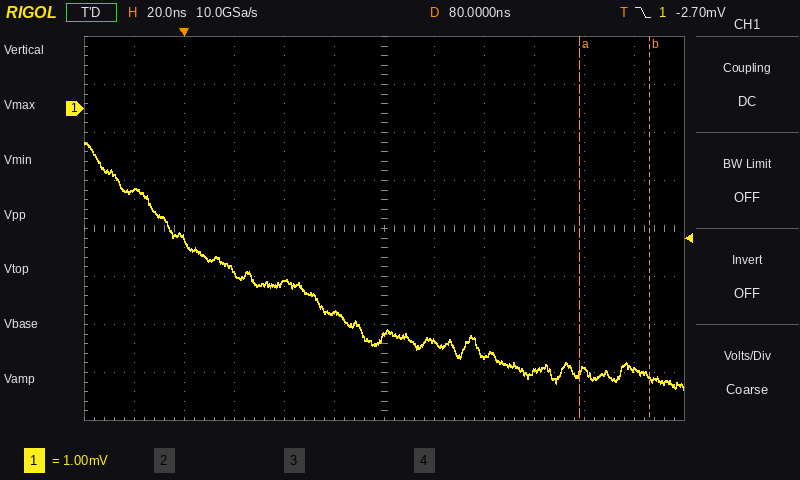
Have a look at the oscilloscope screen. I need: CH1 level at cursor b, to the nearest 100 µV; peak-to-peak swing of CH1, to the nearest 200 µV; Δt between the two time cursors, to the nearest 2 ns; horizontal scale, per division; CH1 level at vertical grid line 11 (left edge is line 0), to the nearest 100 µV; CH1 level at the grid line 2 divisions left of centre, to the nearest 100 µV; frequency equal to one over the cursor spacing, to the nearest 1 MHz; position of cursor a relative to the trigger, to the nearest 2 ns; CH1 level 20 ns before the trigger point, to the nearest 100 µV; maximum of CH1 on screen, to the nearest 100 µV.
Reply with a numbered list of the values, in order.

1. -5.6 mV
2. 5.2 mV
3. 28 ns
4. 20 ns
5. -5.4 mV
6. -3.6 mV
7. 36 MHz
8. +158 ns
9. -1.7 mV
10. -700 µV
